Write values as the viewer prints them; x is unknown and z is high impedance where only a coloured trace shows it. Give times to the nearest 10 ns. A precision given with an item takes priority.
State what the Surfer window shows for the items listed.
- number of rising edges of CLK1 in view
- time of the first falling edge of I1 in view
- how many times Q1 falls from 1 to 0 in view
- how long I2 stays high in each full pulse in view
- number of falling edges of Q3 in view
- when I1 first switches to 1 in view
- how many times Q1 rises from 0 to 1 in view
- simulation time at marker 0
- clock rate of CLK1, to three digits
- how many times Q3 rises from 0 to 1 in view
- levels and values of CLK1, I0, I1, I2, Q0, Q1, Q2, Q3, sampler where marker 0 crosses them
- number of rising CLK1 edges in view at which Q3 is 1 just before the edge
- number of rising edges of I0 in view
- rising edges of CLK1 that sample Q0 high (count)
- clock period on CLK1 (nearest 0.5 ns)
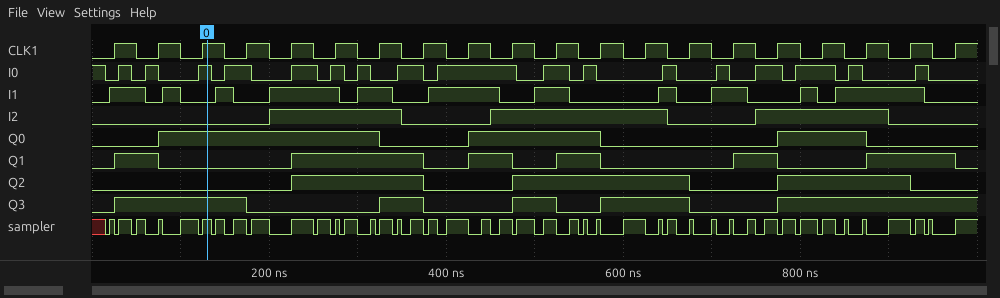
20
60 ns
6
150 ns, 200 ns, 150 ns
4
20 ns
6
130 ns
20.0 MHz
5
CLK1=1, I0=1, I1=0, I2=0, Q0=1, Q1=0, Q2=0, Q3=1, sampler=1
11
17
10
50 ns
